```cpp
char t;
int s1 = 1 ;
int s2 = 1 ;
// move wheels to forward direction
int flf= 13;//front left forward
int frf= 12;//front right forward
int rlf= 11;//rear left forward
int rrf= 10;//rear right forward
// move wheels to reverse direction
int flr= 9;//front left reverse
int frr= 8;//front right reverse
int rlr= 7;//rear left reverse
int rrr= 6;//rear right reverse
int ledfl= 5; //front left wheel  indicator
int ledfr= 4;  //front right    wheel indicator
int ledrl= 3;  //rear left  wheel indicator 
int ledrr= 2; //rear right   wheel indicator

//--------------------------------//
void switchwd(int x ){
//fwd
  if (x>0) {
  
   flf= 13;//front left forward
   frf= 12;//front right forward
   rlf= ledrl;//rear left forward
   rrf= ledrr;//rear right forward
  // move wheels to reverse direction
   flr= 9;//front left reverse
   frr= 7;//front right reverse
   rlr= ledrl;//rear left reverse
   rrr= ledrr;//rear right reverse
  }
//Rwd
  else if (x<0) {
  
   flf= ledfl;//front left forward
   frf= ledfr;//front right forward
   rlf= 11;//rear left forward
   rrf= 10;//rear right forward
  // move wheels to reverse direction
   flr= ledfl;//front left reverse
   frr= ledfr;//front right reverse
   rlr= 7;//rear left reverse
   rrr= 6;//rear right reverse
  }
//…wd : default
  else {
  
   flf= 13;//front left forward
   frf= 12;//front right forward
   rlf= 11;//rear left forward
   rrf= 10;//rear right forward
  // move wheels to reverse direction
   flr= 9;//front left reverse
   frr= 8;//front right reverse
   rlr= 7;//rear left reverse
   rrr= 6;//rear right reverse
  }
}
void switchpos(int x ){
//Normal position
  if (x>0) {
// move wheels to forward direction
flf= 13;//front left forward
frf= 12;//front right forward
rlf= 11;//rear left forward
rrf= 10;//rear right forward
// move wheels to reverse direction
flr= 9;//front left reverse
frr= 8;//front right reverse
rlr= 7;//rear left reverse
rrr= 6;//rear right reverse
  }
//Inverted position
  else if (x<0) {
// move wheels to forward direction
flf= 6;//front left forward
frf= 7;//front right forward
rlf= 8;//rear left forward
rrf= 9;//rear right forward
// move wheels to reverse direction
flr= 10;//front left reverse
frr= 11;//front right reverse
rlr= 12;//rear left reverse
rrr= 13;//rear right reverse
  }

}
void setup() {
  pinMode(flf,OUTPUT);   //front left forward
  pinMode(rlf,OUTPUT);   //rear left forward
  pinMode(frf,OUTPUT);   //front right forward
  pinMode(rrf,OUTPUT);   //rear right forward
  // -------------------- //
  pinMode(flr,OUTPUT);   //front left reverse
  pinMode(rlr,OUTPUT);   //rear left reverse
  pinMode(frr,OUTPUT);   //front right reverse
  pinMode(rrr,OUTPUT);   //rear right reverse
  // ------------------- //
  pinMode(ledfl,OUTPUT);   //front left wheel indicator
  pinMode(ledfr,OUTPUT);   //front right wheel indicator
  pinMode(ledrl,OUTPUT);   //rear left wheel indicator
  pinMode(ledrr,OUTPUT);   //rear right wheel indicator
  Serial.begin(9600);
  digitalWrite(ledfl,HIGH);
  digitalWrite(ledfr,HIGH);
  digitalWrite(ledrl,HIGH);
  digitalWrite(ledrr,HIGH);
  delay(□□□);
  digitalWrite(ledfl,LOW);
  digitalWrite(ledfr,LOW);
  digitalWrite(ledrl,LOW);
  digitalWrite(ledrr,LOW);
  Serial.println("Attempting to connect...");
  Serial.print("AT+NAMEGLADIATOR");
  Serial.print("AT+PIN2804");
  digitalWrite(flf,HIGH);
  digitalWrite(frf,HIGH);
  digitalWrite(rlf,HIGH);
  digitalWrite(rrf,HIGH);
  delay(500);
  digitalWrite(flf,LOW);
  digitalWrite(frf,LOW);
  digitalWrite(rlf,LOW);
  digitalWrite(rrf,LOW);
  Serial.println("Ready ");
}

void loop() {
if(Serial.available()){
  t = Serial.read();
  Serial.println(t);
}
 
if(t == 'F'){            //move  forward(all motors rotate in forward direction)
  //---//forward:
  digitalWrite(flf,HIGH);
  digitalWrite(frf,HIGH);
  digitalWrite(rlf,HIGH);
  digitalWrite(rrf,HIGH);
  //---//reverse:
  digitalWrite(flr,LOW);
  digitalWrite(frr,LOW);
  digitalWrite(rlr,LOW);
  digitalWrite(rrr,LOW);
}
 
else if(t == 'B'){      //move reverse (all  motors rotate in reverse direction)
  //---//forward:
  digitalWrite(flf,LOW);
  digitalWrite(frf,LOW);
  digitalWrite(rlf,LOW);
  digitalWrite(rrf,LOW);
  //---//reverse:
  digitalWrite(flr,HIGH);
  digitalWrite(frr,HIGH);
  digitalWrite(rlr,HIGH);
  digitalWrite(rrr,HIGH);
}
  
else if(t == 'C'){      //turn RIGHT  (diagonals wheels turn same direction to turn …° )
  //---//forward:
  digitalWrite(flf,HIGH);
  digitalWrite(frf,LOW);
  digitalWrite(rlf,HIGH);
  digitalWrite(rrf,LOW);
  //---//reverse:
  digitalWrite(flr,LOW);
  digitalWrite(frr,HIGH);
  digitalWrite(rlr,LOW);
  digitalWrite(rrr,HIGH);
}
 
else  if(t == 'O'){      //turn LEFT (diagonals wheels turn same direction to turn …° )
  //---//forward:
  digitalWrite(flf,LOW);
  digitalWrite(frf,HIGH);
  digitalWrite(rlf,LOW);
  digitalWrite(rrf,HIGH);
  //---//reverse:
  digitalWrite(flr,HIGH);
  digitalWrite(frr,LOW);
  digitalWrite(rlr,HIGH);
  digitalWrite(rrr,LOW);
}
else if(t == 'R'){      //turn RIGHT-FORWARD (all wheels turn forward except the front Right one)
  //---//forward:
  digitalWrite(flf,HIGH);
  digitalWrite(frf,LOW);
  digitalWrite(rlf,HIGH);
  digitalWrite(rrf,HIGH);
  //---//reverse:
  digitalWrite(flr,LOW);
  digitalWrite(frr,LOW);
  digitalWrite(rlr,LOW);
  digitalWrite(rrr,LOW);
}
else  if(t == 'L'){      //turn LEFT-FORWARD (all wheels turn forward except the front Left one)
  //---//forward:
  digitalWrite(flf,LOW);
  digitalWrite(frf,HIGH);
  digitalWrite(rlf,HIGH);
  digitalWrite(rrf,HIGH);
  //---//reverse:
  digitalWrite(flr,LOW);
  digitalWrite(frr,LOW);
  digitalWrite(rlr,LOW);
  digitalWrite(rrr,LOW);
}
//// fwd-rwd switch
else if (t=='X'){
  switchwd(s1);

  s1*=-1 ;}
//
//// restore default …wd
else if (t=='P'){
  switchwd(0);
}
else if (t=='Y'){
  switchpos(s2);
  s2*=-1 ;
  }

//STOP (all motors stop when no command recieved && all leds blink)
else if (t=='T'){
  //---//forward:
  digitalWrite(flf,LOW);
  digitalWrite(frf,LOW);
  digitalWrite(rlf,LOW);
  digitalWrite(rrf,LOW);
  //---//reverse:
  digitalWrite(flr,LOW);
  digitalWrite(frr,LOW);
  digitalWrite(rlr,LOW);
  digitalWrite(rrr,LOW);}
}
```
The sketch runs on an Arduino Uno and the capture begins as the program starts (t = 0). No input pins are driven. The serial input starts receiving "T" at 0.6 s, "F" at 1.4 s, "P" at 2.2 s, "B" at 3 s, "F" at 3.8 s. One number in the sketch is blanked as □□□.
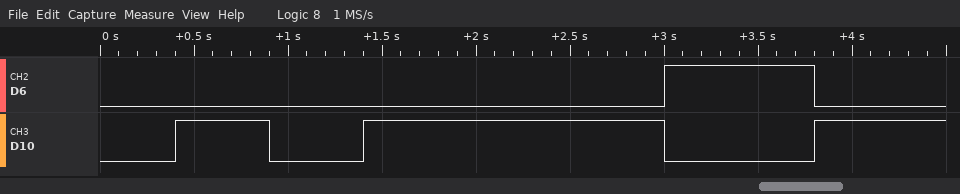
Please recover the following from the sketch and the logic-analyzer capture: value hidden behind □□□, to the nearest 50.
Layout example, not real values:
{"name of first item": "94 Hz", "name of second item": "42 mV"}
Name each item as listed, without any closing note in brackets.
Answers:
{"value hidden behind □□□, to the nearest 50": "400"}
